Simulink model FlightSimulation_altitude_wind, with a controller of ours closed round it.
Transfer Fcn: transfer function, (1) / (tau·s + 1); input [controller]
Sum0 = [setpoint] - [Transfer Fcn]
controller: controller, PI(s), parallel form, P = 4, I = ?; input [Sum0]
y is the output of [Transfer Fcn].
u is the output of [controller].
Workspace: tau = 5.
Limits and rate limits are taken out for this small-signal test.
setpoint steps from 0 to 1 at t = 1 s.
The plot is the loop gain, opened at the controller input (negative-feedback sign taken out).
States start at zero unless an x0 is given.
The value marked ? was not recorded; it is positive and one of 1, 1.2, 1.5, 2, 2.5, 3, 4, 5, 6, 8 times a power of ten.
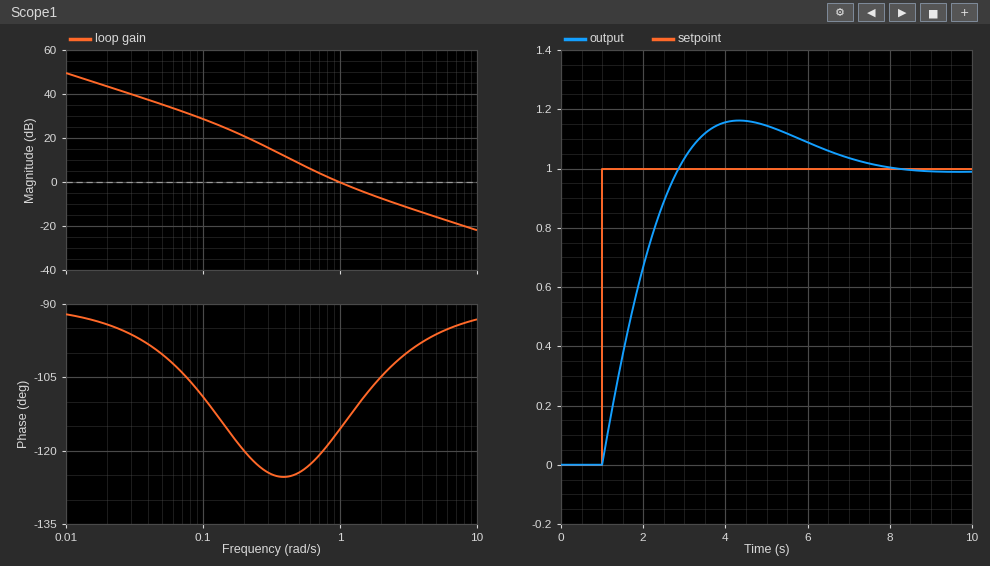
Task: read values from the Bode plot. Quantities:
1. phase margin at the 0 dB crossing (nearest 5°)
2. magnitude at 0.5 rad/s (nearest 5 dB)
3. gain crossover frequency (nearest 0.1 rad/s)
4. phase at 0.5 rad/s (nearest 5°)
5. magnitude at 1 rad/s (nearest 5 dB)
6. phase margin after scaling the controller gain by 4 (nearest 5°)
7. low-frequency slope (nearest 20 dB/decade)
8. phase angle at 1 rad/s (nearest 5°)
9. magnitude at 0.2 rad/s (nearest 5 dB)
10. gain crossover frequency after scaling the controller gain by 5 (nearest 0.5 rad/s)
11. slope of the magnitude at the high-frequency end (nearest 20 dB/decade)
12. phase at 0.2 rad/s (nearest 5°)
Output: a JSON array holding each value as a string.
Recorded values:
["65°", "10 dB", "1.0 rad/s", "-125°", "0 dB", "80°", "-20 dB/decade", "-115°", "20 dB", "4.0 rad/s", "-20 dB/decade", "-120°"]
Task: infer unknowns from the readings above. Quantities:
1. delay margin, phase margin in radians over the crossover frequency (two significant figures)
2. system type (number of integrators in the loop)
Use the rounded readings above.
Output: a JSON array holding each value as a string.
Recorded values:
["1.1 s", "1"]
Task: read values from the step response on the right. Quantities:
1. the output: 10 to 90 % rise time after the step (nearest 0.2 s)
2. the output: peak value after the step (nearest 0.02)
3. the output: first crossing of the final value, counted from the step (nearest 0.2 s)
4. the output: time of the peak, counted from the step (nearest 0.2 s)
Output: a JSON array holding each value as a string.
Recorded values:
["1.4 s", "1.16", "1.8 s", "3.4 s"]
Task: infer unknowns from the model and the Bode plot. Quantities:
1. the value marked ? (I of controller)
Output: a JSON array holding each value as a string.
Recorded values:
["3"]
